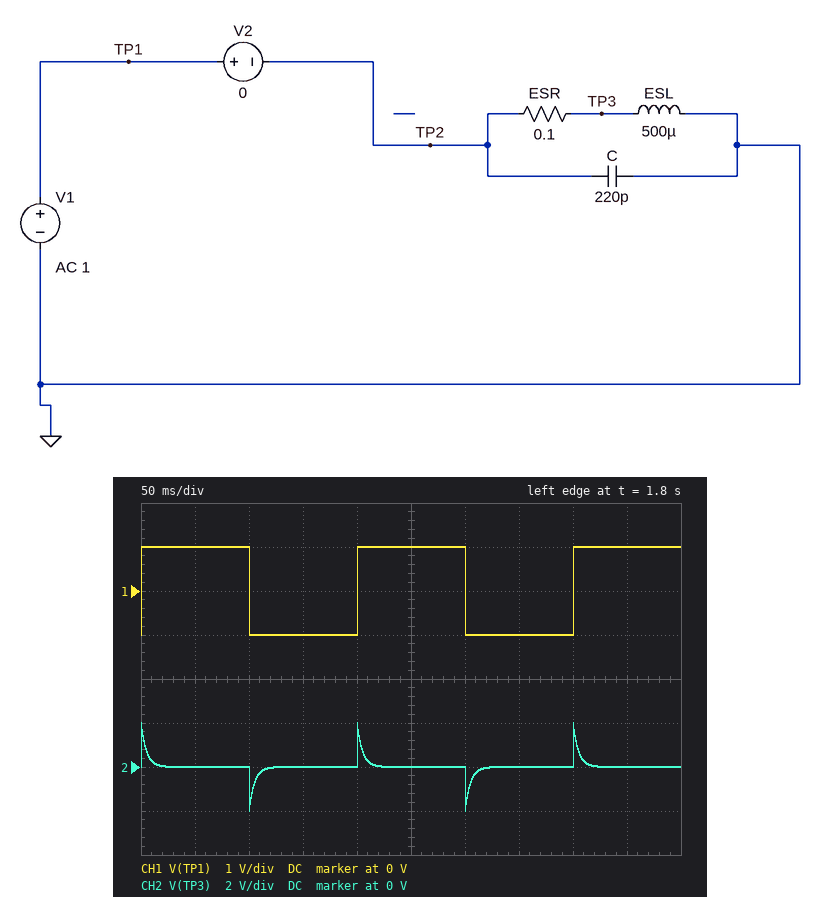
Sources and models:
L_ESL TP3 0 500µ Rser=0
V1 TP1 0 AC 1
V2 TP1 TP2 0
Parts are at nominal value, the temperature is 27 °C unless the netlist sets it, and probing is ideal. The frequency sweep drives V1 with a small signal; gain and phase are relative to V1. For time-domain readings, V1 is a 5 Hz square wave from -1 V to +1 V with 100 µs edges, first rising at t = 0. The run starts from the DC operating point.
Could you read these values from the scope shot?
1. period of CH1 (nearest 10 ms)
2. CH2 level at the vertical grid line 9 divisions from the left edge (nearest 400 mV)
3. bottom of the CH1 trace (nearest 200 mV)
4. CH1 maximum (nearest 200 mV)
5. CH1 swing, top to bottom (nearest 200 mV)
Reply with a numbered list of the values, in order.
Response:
1. 200 ms
2. 0 V
3. -1.0 V
4. 1.0 V
5. 2.0 V
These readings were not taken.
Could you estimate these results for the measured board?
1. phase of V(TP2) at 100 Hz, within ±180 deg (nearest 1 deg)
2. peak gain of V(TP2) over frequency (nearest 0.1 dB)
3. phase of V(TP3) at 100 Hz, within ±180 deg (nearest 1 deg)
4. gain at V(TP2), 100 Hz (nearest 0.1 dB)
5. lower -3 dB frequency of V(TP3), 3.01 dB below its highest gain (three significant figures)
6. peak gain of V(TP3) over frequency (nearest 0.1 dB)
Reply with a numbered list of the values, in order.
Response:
1. 0 deg
2. 0 dB
3. 18 deg
4. 0 dB
5. 31.8 Hz
6. 0 dB
